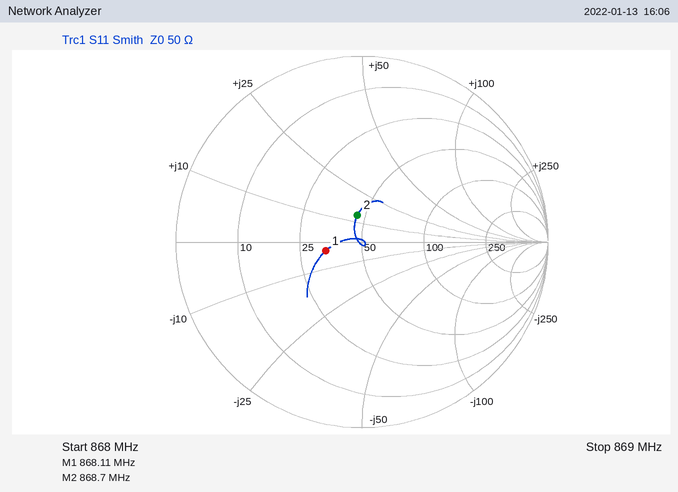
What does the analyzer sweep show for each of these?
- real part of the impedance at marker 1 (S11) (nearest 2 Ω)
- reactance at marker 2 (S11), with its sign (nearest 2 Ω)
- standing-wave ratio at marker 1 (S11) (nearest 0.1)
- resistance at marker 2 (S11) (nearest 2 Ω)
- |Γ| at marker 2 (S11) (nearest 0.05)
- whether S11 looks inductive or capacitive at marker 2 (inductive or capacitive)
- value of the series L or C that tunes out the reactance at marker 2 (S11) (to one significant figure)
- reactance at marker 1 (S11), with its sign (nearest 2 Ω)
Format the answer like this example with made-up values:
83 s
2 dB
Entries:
34 Ω
+14 Ω
1.5
46 Ω
0.15
inductive
10 pF
-4 Ω
